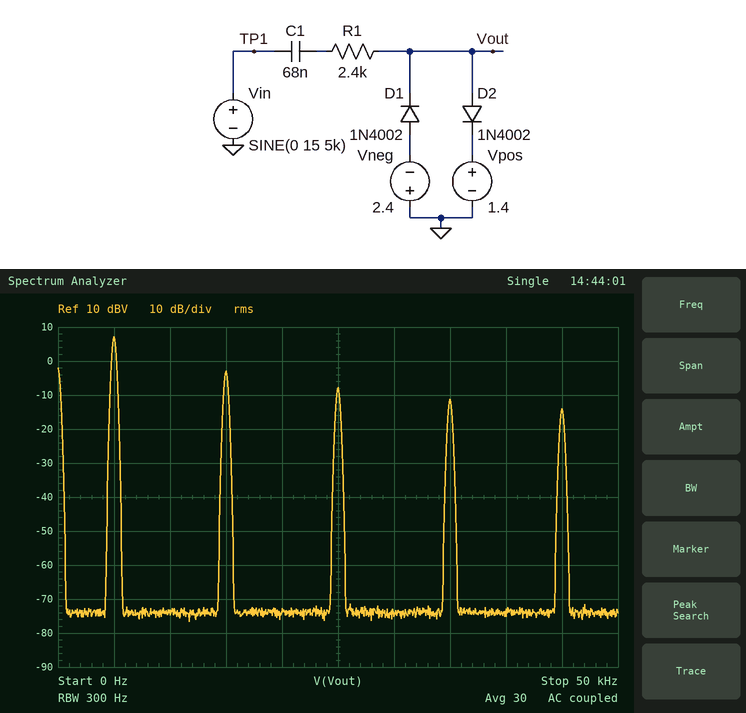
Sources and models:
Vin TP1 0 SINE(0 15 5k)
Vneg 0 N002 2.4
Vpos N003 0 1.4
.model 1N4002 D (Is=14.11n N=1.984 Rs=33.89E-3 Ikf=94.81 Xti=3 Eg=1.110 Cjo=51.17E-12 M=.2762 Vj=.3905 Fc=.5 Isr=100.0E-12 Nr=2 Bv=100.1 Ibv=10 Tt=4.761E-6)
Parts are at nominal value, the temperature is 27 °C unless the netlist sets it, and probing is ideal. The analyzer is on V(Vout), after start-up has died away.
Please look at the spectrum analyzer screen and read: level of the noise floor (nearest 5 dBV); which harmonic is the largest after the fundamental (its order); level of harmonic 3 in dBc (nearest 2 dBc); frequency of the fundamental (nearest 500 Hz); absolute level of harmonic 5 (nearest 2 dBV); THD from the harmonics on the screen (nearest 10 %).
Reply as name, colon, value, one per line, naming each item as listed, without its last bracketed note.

level of the noise floor: -75 dBV
which harmonic is the largest after the fundamental: 3
level of harmonic 3 in dBc: -10 dBc
frequency of the fundamental: 5.0 kHz
absolute level of harmonic 5: -8 dBV
THD from the harmonics on the screen: 40 %
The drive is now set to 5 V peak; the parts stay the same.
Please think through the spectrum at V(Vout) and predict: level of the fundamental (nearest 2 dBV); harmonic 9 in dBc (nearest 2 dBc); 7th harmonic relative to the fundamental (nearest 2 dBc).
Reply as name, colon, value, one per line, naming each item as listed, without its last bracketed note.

level of the fundamental: 6 dBV
harmonic 9 in dBc: -32 dBc
7th harmonic relative to the fundamental: -40 dBc
